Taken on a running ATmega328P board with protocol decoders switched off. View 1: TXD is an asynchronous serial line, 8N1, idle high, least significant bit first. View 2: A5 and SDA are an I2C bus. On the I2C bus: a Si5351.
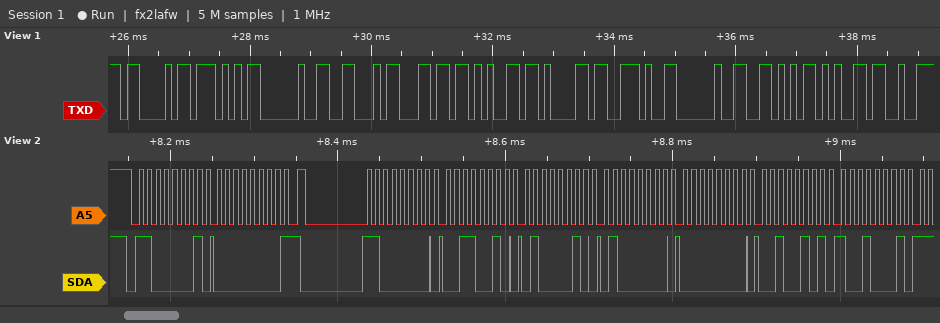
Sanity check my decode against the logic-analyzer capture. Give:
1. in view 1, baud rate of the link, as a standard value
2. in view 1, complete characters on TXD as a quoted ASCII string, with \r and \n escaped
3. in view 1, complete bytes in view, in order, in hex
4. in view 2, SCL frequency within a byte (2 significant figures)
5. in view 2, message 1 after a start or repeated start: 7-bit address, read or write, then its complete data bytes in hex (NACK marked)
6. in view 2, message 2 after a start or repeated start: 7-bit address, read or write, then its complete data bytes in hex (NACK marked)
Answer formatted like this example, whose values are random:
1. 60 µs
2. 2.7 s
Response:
1. 9600 baud
2. "CW Flea. Ve"
3. 43 57 20 46 6C 65 61 2E 20 56 65
4. 100 kHz
5. 0x60 read: 00 NACK
6. 0x60 write: 32 42 40 00 25 91
